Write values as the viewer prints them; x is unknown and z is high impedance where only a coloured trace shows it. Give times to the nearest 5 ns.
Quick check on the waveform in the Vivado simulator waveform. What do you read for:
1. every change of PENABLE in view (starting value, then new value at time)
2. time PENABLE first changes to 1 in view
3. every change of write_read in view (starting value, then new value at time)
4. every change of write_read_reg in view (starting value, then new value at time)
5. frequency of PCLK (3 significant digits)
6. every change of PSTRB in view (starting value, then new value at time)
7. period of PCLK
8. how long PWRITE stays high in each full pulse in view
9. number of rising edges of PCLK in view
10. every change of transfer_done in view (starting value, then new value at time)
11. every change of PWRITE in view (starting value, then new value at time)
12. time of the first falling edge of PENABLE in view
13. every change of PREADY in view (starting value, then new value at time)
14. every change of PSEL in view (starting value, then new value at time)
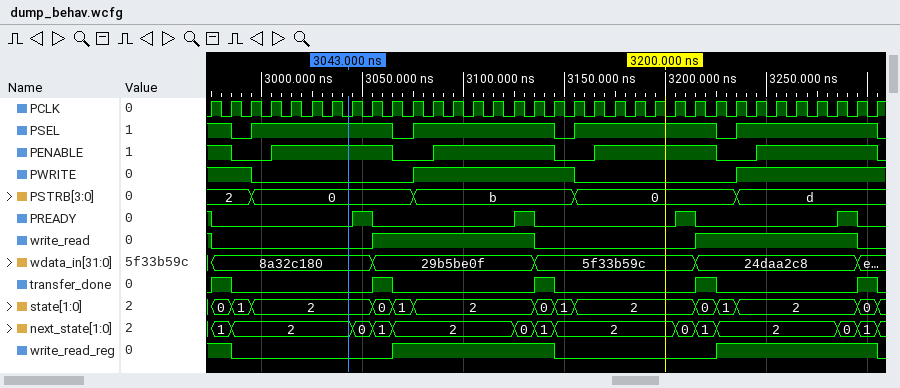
1, 0 at 2985 ns, 1 at 3005 ns, 0 at 3065 ns, 1 at 3085 ns, 0 at 3145 ns, 1 at 3165 ns, 0 at 3225 ns, 1 at 3245 ns, 0 at 3305 ns
3005 ns
1, 0 at 2975 ns, 1 at 3055 ns, 0 at 3135 ns, 1 at 3215 ns, 0 at 3295 ns
1, 0 at 2985 ns, 1 at 3065 ns, 0 at 3145 ns, 1 at 3225 ns, 0 at 3305 ns
100 MHz
2, 0 at 2995 ns, b at 3075 ns, 0 at 3155 ns, d at 3235 ns
10 ns
80 ns
34
0, 1 at 2975 ns, 0 at 2985 ns, 1 at 3055 ns, 0 at 3065 ns, 1 at 3135 ns, 0 at 3145 ns, 1 at 3215 ns, 0 at 3225 ns, 1 at 3295 ns, 0 at 3305 ns
1, 0 at 2995 ns, 1 at 3075 ns, 0 at 3155 ns, 1 at 3235 ns
2985 ns
1, 0 at 2975 ns, 1 at 3045 ns, 0 at 3055 ns, 1 at 3125 ns, 0 at 3135 ns, 1 at 3205 ns, 0 at 3215 ns, 1 at 3285 ns, 0 at 3295 ns
1, 0 at 2985 ns, 1 at 2995 ns, 0 at 3065 ns, 1 at 3075 ns, 0 at 3145 ns, 1 at 3155 ns, 0 at 3225 ns, 1 at 3235 ns, 0 at 3305 ns
